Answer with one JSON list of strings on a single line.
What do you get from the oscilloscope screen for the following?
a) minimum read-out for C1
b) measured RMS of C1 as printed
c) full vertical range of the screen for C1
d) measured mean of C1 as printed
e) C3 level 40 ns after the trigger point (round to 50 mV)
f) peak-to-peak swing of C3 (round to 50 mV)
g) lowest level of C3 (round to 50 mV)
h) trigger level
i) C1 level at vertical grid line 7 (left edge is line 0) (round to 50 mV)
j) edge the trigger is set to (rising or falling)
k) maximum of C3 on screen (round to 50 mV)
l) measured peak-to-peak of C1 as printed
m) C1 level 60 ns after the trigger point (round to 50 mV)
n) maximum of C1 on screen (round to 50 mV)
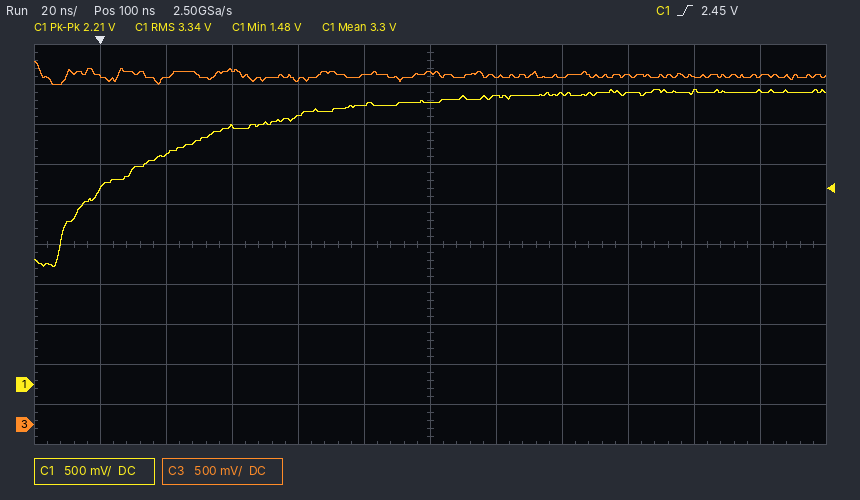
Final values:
["1.48 V", "3.34 V", "5 V", "3.3 V", "4.45 V", "300 mV", "4.25 V", "2.45 V", "3.60 V", "rising", "4.55 V", "2.21 V", "3.35 V", "3.70 V"]
